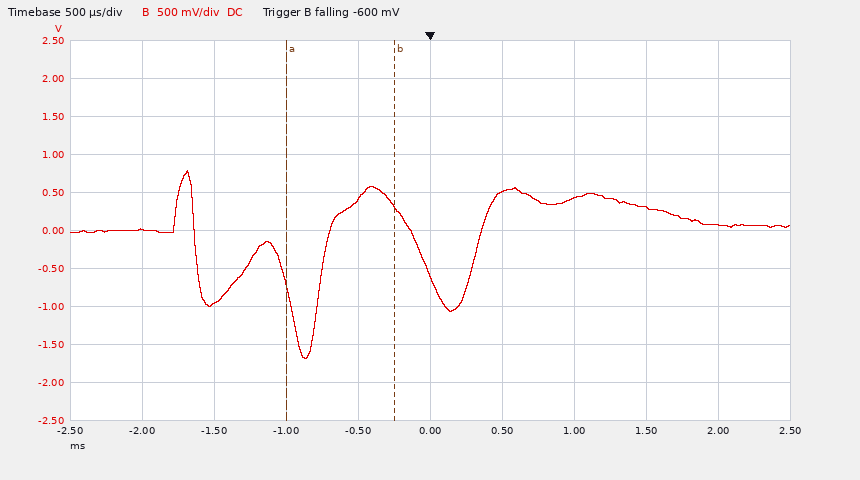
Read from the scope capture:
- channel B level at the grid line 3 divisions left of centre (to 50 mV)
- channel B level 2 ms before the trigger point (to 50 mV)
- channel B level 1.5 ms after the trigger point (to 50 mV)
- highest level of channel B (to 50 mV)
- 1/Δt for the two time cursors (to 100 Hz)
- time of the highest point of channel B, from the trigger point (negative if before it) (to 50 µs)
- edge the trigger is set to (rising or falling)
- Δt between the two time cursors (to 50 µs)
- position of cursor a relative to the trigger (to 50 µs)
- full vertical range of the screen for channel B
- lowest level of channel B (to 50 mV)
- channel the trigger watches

-950 mV
0 mV
300 mV
800 mV
1.3 kHz
-1.70 ms
falling
750 µs
-1.00 ms
5 V
-1.70 V
channel B
